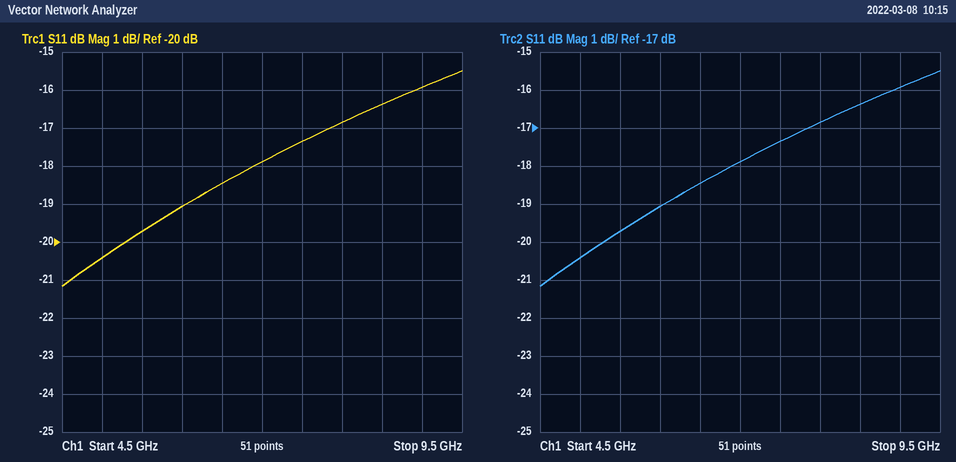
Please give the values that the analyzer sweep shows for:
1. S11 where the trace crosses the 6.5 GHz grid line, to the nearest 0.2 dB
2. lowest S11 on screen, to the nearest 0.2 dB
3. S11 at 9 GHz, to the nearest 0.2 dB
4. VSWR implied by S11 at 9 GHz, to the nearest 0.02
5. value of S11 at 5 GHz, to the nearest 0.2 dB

-18.4 dB
-21.2 dB
-16.0 dB
1.38
-20.4 dB
